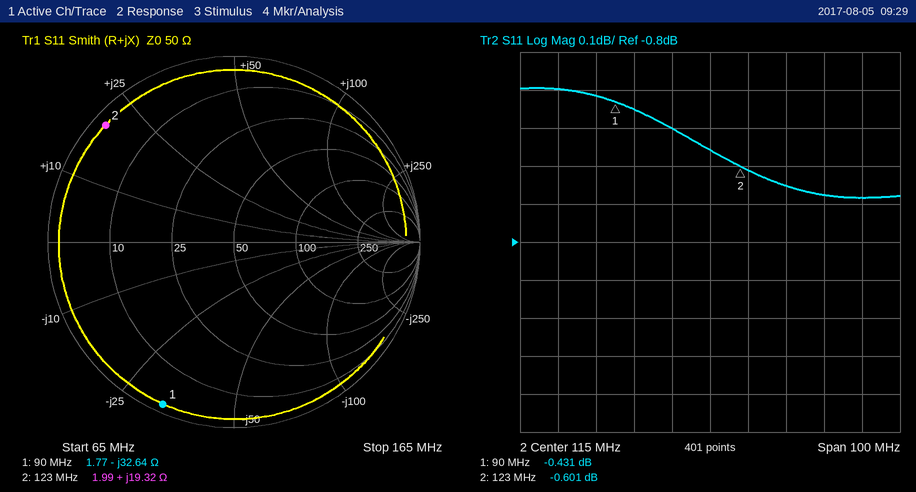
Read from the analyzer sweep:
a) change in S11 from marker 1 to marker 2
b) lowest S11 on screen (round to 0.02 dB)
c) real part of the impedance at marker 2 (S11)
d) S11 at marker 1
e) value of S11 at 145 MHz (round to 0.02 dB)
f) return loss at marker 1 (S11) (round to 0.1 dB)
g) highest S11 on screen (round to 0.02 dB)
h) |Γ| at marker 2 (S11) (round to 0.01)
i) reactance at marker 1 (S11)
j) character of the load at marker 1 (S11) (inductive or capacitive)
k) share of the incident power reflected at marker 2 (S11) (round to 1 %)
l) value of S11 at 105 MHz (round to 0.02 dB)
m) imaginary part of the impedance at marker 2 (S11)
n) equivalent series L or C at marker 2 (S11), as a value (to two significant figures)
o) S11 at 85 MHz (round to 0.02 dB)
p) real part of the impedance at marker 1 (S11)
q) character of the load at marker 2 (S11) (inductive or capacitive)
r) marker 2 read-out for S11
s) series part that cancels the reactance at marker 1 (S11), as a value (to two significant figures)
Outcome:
-0.170 dB
-0.68 dB
1.99 Ω
-0.431 dB
-0.68 dB
0.4 dB
-0.40 dB
0.93
-32.64 Ω
capacitive
87 %
-0.50 dB
+19.32 Ω
25 nH
-0.42 dB
1.77 Ω
inductive
-0.601 dB
58 nH
